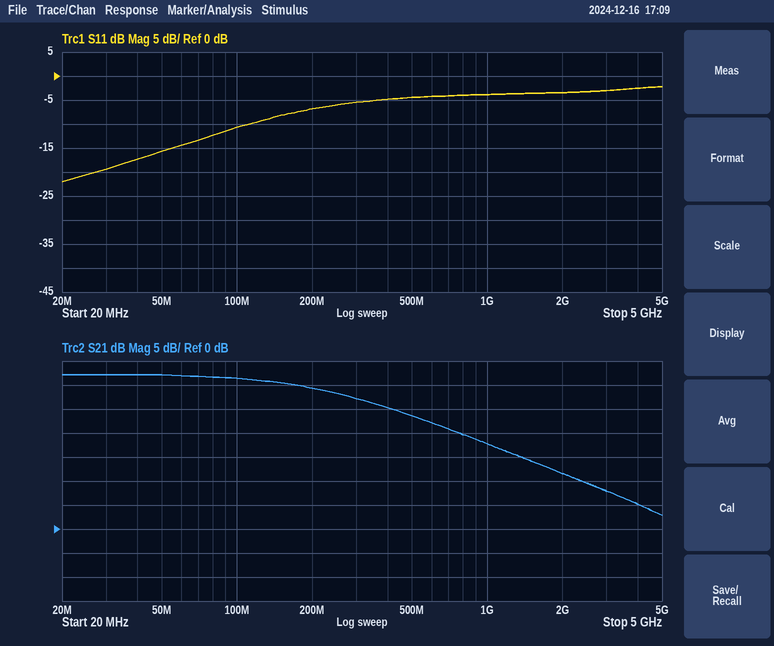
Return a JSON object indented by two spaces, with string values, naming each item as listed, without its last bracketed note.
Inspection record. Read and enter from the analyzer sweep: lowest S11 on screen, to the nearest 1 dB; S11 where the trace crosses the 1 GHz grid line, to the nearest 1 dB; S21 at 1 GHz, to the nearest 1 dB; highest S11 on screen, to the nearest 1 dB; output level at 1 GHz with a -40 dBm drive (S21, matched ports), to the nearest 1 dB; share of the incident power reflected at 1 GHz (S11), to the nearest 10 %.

{
  "lowest S11 on screen, to the nearest 1 dB": "-22 dB",
  "S11 where the trace crosses the 1 GHz grid line, to the nearest 1 dB": "-4 dB",
  "S21 at 1 GHz, to the nearest 1 dB": "18 dB",
  "highest S11 on screen, to the nearest 1 dB": "-2 dB",
  "output level at 1 GHz with a -40 dBm drive (S21, matched ports), to the nearest 1 dB": "-22 dBm",
  "share of the incident power reflected at 1 GHz (S11), to the nearest 10 %": "40 %"
}
